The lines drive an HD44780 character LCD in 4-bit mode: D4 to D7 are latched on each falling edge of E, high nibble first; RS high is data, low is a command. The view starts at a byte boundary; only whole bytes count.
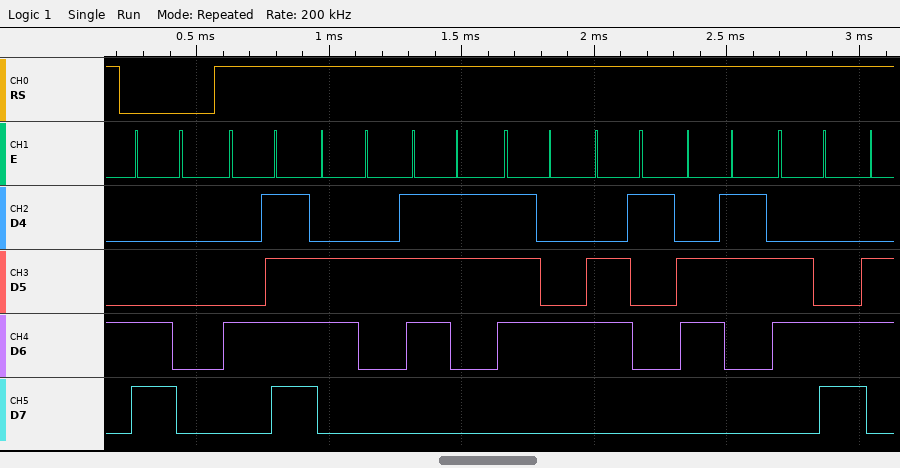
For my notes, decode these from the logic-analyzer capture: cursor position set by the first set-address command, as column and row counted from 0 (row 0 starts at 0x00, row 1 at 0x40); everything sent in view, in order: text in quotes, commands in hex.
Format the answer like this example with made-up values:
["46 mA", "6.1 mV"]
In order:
["column 0, row 1", "0xC0 \"Obstacl\""]
